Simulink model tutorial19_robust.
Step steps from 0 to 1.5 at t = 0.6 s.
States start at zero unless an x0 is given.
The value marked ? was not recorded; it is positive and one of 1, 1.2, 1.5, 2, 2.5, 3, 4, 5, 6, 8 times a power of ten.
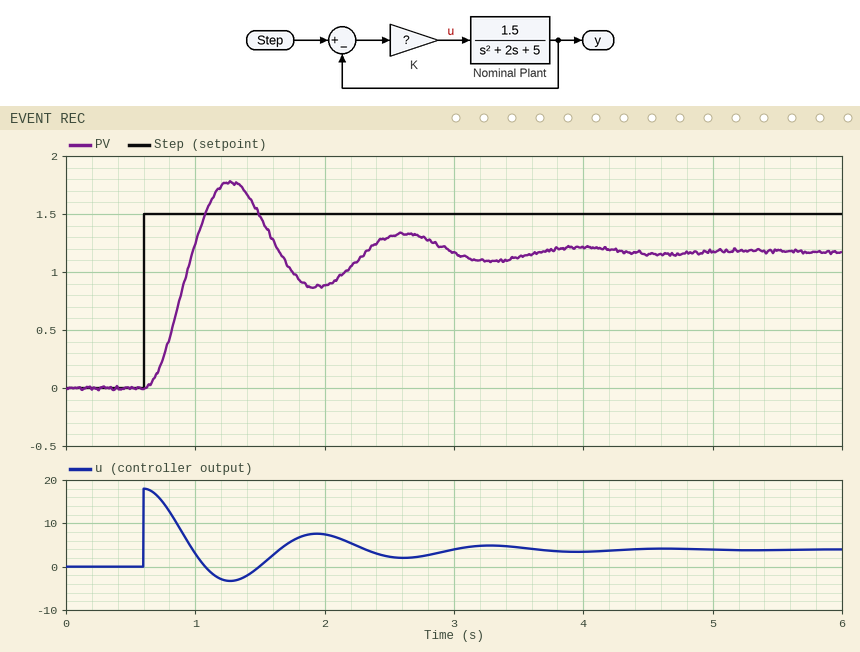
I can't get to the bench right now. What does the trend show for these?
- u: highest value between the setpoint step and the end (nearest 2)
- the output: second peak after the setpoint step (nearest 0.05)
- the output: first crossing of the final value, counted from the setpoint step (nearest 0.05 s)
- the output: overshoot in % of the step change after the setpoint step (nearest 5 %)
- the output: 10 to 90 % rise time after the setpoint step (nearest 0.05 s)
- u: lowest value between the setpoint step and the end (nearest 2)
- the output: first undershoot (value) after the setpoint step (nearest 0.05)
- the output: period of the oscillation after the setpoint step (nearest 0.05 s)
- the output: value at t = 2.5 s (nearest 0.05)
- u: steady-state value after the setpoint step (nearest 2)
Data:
18
1.35
0.40 s
50 %
0.25 s
-4
0.85
1.35 s
1.30
4
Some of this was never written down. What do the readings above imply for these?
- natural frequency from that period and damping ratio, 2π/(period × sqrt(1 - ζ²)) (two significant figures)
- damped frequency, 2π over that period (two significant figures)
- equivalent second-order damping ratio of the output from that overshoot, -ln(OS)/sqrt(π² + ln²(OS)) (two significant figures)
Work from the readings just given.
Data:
4.8 rad/s
4.7 rad/s
0.22
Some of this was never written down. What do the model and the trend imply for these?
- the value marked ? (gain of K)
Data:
12
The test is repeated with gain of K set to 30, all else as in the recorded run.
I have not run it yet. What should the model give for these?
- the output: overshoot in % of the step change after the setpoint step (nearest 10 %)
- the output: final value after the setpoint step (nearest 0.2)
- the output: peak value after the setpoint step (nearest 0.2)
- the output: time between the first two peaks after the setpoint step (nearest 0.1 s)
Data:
60 %
1.4
2.2
0.9 s
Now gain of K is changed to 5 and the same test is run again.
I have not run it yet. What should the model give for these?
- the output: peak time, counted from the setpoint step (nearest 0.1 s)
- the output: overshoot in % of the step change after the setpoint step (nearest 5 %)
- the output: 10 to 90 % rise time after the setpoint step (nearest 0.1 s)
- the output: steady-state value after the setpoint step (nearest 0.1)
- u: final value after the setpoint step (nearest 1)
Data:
0.9 s
40 %
0.4 s
0.9
3
